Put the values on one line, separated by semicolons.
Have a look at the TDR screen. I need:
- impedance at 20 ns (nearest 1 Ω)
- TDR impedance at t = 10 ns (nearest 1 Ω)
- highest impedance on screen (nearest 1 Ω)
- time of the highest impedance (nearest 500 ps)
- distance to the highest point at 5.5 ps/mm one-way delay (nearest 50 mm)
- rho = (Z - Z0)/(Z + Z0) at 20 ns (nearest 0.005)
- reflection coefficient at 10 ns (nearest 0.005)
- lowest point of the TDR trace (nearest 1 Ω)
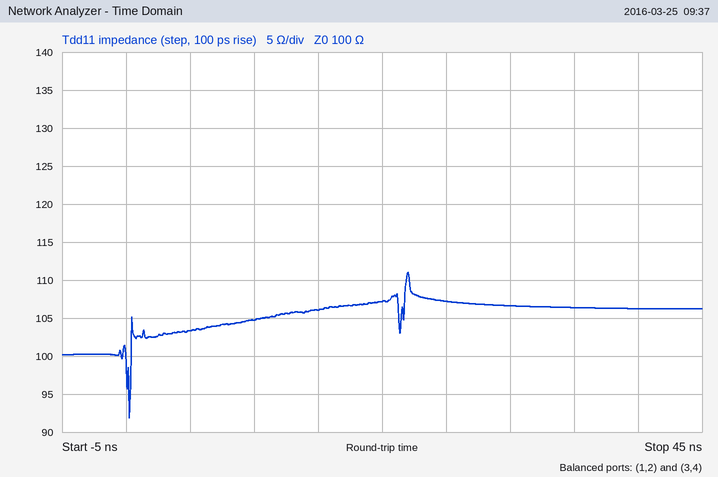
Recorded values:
107 Ω; 105 Ω; 111 Ω; 22.0 ns; 2.00 m; +0.035; +0.025; 92 Ω
